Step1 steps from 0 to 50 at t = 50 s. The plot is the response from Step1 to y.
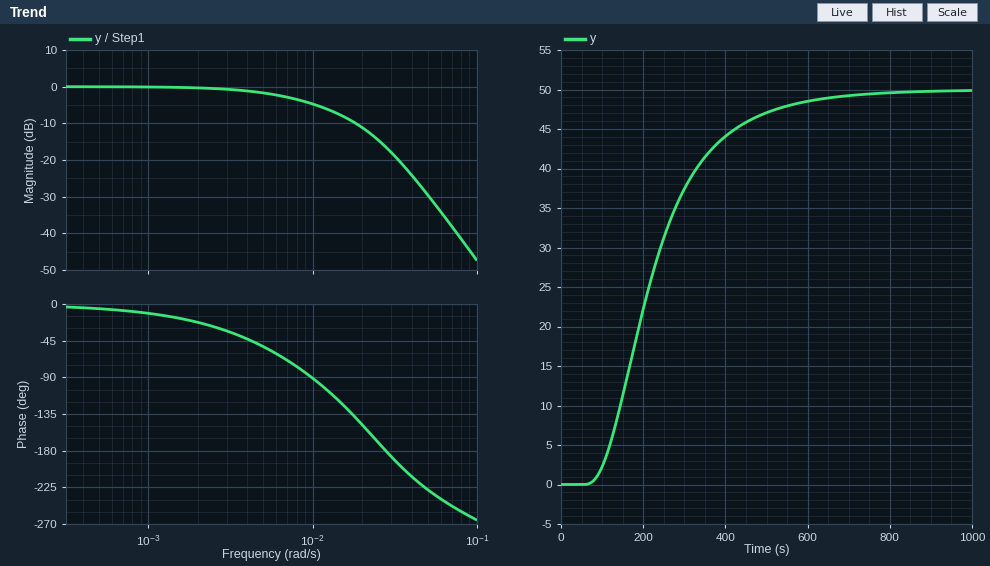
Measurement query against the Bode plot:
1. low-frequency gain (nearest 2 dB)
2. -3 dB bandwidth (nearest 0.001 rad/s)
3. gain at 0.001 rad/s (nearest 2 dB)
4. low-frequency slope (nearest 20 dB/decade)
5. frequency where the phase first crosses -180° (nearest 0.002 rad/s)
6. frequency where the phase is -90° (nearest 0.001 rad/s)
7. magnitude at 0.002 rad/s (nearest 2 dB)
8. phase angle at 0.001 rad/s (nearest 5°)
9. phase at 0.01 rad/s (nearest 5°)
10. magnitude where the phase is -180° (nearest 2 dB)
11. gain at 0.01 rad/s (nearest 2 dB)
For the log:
0 dB
0.007 rad/s
0 dB
0 dB/decade
0.028 rad/s
0.010 rad/s
0 dB
-10°
-90°
-16 dB
-4 dB
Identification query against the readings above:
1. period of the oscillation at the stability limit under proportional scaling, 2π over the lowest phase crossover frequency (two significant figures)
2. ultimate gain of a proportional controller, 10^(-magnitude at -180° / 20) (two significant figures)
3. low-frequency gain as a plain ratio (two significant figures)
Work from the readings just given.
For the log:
220 s
6.3
1.0
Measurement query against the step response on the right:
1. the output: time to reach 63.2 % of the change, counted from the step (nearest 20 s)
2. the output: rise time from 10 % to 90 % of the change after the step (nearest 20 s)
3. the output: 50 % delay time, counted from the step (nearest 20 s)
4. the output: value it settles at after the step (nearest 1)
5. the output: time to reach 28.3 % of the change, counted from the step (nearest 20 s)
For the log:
200 s
300 s
160 s
50
120 s
